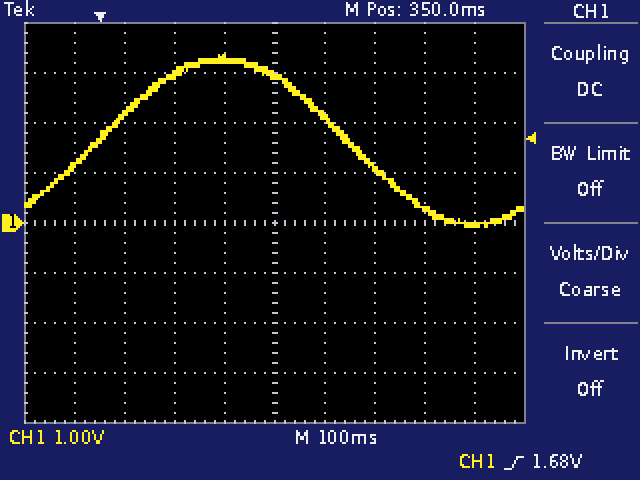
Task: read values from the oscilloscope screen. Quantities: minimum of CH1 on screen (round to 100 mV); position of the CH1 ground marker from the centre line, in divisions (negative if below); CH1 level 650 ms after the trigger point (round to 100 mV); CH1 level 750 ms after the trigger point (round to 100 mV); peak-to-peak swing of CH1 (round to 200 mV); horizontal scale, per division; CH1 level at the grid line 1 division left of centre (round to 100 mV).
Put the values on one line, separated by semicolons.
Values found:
-100 mV; 0.0 div; 300 mV; 0.0 V; 3.4 V; 100 ms; 3.3 V
